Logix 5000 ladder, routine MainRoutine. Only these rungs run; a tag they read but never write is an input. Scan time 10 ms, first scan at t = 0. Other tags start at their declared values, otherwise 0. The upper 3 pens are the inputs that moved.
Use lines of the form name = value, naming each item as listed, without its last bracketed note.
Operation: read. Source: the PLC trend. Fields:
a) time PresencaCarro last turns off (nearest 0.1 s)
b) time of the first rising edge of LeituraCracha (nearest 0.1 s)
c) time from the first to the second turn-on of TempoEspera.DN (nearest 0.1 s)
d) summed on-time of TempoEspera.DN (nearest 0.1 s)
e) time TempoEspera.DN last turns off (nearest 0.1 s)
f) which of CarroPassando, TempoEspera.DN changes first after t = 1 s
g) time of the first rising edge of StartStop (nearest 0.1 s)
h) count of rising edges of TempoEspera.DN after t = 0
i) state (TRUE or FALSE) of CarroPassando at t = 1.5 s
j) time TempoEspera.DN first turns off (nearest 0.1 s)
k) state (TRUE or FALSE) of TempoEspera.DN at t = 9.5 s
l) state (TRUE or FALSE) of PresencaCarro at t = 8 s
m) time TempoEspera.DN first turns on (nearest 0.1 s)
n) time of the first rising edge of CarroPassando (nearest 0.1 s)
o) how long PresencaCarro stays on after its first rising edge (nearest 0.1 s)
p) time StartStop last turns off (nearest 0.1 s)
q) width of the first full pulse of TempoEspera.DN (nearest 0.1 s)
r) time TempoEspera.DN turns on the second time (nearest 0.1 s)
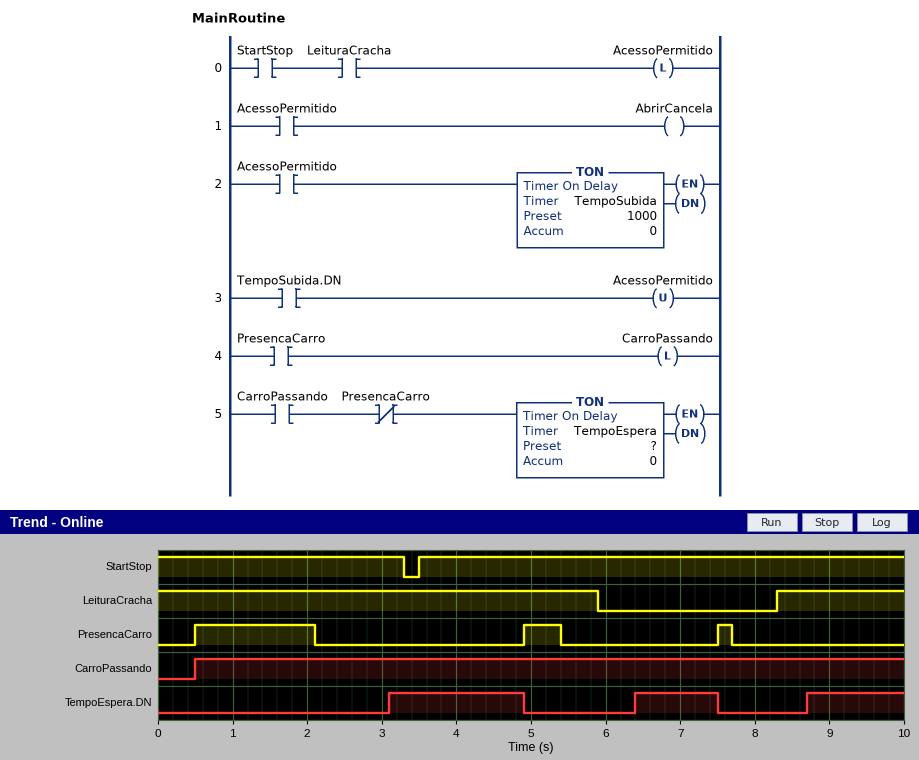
time PresencaCarro last turns off = 7.7 s
time of the first rising edge of LeituraCracha = 8.3 s
time from the first to the second turn-on of TempoEspera.DN = 3.3 s
summed on-time of TempoEspera.DN = 4.2 s
time TempoEspera.DN last turns off = 7.5 s
which of CarroPassando, TempoEspera.DN changes first after t = 1 s = TempoEspera.DN
time of the first rising edge of StartStop = 3.5 s
count of rising edges of TempoEspera.DN after t = 0 = 3
state (TRUE or FALSE) of CarroPassando at t = 1.5 s = TRUE
time TempoEspera.DN first turns off = 4.9 s
state (TRUE or FALSE) of TempoEspera.DN at t = 9.5 s = TRUE
state (TRUE or FALSE) of PresencaCarro at t = 8 s = FALSE
time TempoEspera.DN first turns on = 3.1 s
time of the first rising edge of CarroPassando = 0.5 s
how long PresencaCarro stays on after its first rising edge = 1.6 s
time StartStop last turns off = 3.3 s
width of the first full pulse of TempoEspera.DN = 1.8 s
time TempoEspera.DN turns on the second time = 6.4 s
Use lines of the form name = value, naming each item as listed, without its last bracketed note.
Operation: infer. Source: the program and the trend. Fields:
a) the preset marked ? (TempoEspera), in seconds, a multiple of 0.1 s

the preset marked ? (TempoEspera), in seconds, a multiple of 0.1 s = 1.0 s
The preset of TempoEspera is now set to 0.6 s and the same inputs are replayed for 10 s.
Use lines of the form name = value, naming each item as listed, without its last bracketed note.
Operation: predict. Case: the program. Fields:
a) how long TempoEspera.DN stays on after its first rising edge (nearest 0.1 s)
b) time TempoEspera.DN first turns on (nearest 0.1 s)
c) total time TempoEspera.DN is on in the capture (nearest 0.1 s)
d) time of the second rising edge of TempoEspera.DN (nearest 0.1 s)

how long TempoEspera.DN stays on after its first rising edge = 2.2 s
time TempoEspera.DN first turns on = 2.7 s
total time TempoEspera.DN is on in the capture = 5.4 s
time of the second rising edge of TempoEspera.DN = 6.0 s
